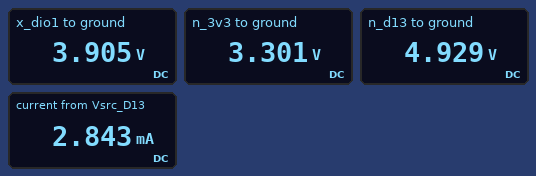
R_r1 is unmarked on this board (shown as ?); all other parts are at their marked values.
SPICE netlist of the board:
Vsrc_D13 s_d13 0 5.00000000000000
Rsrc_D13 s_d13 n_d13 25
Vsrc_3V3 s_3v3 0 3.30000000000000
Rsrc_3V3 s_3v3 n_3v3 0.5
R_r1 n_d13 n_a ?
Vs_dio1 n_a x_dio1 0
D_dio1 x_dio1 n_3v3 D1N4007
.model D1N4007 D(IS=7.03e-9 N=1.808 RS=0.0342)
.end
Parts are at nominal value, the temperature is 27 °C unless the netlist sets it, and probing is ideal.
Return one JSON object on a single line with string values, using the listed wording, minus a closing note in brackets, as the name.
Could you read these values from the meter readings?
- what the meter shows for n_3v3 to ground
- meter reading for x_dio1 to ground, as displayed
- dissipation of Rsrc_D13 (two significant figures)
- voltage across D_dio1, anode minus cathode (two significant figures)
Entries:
{"what the meter shows for n_3v3 to ground": "3.301 V", "meter reading for x_dio1 to ground, as displayed": "3.905 V", "dissipation of Rsrc_D13": "200 µW", "voltage across D_dio1, anode minus cathode": "600 mV"}
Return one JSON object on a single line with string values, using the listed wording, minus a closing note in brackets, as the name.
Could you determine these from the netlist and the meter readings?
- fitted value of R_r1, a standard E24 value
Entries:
{"fitted value of R_r1, a standard E24 value": "360 Ω"}
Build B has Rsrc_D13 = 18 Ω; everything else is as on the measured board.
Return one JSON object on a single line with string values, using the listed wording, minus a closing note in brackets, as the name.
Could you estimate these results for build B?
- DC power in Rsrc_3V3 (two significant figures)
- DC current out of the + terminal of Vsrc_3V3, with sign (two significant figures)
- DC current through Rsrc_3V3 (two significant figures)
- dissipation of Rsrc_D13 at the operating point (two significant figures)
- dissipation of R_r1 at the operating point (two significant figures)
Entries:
{"DC power in Rsrc_3V3": "4.2 µW", "DC current out of the + terminal of Vsrc_3V3, with sign": "-2.9 mA", "DC current through Rsrc_3V3": "2.9 mA", "dissipation of Rsrc_D13 at the operating point": "150 µW", "dissipation of R_r1 at the operating point": "3.0 mW"}
